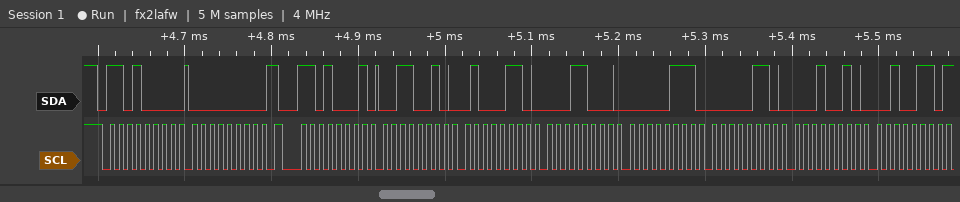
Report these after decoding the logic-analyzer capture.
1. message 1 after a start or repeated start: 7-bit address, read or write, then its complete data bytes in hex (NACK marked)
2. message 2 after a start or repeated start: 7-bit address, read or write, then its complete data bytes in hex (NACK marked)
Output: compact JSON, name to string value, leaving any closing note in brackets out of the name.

{"message 1 after a start or repeated start: 7-bit address, read or write, then its complete data bytes in hex": "0x68 write: 00", "message 2 after a start or repeated start: 7-bit address, read or write, then its complete data bytes in hex": "0x68 read: 32 46 18 07 06 12 26 NACK"}
